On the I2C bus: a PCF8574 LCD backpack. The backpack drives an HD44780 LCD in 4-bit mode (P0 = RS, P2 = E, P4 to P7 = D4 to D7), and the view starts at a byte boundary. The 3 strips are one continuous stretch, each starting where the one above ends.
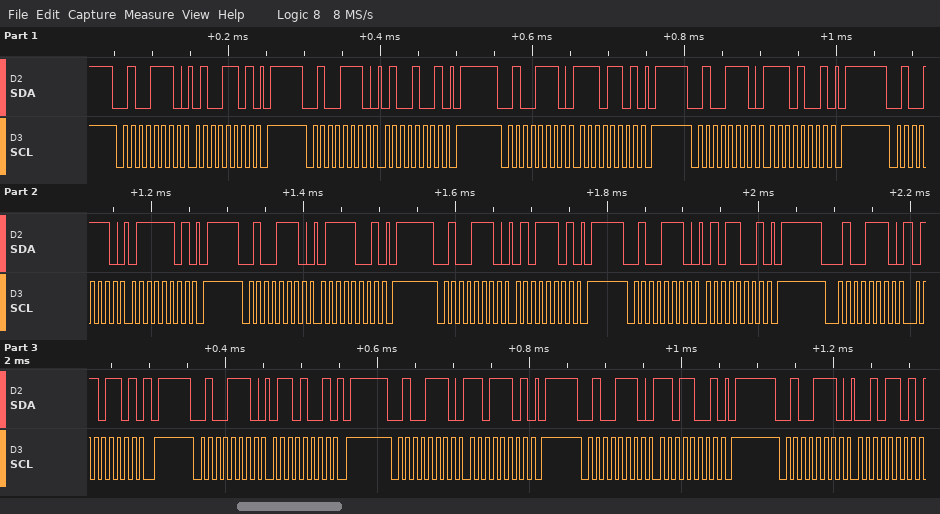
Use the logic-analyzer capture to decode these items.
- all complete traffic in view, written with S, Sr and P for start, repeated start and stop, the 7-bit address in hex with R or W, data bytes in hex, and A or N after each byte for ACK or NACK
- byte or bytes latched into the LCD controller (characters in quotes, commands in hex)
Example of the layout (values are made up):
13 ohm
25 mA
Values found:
S 27W A 4D A P S 27W A 49 A P S 27W A ED A P S 27W A E9 A P S 27W A 7D A P S 27W A 79 A P S 27W A 5D A P S 27W A 59 A P S 27W A 6D A P S 27W A 69 A P S 27W A DD A P S 27W A D9 A P S 27W A 2D A
'N' 'u' 'm'
